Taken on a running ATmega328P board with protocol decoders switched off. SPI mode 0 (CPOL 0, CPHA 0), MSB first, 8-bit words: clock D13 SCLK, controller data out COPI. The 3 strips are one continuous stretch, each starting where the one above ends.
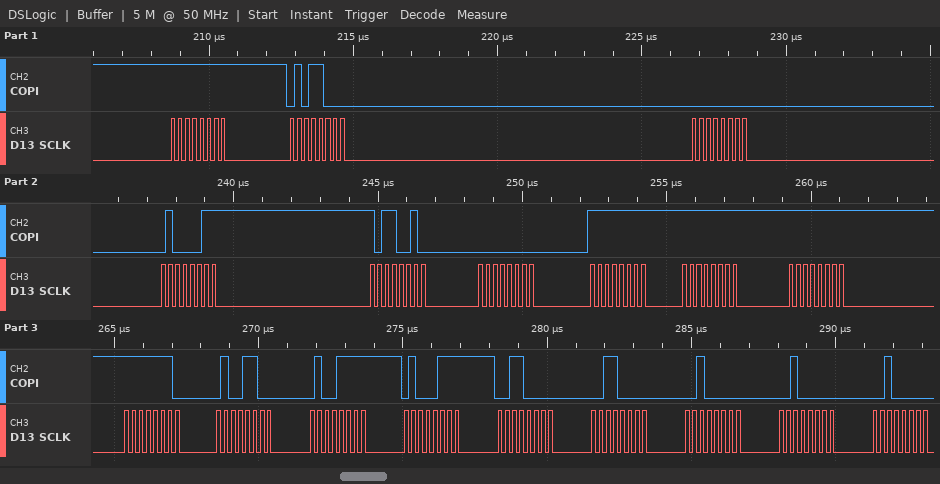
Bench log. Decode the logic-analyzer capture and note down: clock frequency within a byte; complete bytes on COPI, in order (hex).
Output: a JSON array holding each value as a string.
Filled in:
["4 MHz", "FF 58 00 43 B2 00 FF FF FF FE 4C 4F 47 30 30 20 20 20"]
